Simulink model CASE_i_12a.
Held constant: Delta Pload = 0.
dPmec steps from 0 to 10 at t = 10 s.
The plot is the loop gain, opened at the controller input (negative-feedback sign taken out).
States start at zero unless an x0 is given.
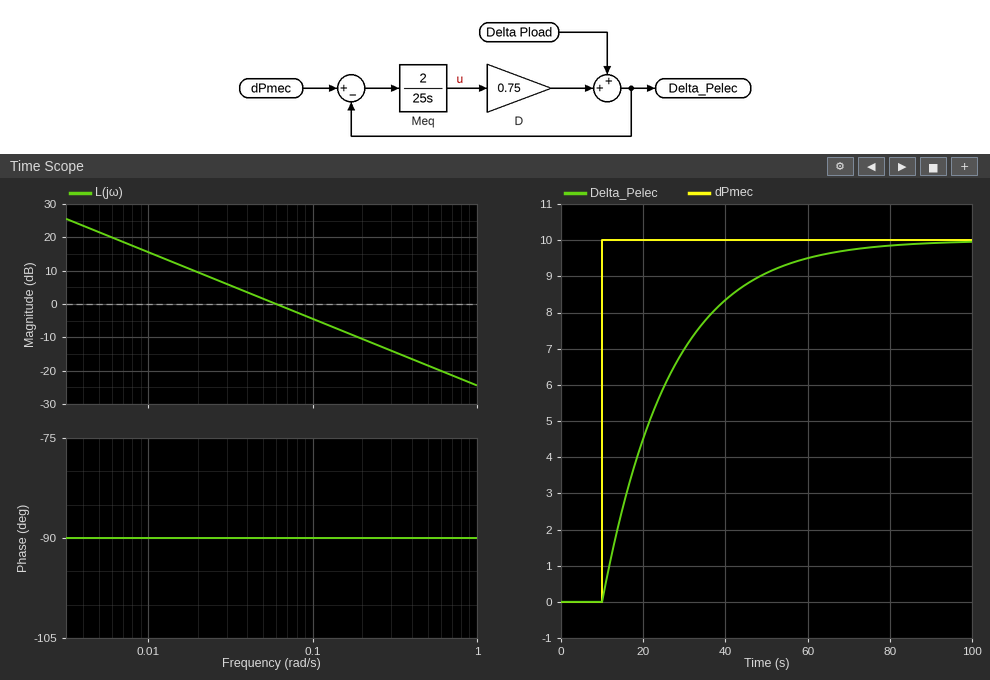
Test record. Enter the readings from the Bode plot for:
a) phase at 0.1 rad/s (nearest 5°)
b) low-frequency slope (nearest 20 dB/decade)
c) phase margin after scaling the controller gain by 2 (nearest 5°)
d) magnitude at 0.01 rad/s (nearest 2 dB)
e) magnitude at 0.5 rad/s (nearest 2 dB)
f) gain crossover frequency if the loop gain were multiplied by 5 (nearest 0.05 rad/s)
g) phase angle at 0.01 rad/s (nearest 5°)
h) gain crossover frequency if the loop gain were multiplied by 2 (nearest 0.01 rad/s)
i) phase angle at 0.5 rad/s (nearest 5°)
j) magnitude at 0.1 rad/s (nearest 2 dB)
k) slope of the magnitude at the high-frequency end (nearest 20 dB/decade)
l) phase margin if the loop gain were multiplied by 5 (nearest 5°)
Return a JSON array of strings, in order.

["-90°", "-20 dB/decade", "90°", "16 dB", "-18 dB", "0.30 rad/s", "-90°", "0.12 rad/s", "-90°", "-4 dB", "-20 dB/decade", "90°"]
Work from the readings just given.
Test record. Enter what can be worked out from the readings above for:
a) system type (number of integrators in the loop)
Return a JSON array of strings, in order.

["1"]
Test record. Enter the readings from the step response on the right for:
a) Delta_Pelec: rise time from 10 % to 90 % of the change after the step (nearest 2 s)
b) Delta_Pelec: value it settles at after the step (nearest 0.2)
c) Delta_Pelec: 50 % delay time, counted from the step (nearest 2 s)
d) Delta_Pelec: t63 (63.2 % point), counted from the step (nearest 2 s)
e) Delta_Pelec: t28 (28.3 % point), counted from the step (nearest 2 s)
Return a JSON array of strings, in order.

["36 s", "10.0", "12 s", "16 s", "6 s"]
